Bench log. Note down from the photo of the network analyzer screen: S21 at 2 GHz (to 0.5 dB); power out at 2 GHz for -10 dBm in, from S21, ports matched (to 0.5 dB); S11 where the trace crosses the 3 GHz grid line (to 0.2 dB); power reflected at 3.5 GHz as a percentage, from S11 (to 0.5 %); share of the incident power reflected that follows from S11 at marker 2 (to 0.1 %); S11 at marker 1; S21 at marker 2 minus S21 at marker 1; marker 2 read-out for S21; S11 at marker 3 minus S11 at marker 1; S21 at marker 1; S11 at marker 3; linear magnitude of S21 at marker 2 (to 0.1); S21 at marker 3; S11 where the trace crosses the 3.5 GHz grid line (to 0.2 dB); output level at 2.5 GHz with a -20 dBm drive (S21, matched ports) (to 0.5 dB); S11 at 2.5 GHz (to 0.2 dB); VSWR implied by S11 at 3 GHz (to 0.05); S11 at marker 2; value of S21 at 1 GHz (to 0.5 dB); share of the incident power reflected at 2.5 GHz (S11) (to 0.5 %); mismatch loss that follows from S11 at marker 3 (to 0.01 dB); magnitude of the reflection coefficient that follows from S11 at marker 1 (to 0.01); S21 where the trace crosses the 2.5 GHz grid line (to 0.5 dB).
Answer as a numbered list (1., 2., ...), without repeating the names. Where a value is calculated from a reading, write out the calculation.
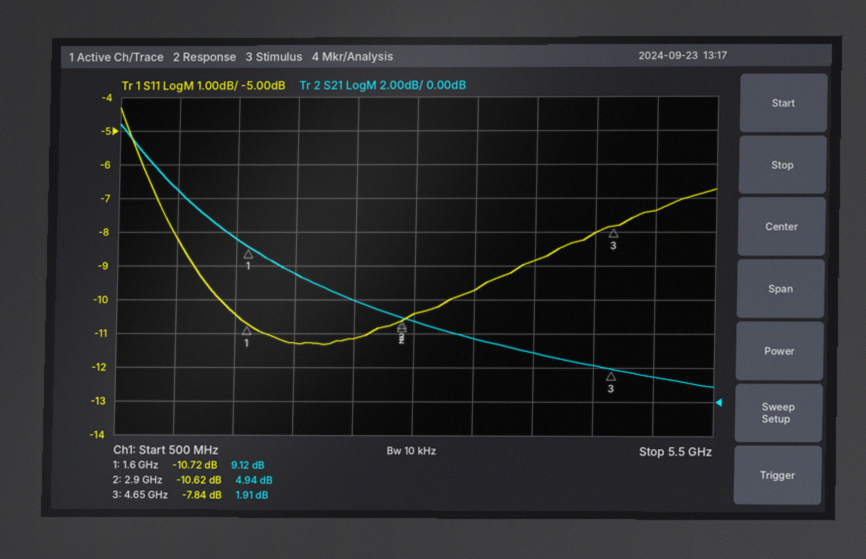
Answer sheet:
1. 7.5 dB
2. -10 dBm + (7.5 dB) = -2.5 dBm
3. -10.4 dB
4. 10^(-9.8/10) ≈ 10.5 %
5. 10^(-10.62/10) ≈ 8.7 %
6. -10.72 dB
7. 4.94 − (9.12) = -4.18 dB
8. 4.94 dB
9. -7.84 − (-10.72) = 2.88 dB
10. 9.12 dB
11. -7.84 dB
12. 10^(4.94/20) ≈ 1.8
13. 1.91 dB
14. -9.8 dB
15. -20 dBm + (6.0 dB) = -14.0 dBm
16. -11.2 dB
17. |Γ| = 10^(-10.4/20) = 0.3020; VSWR = (1 + 0.3020)/(1 − 0.3020) ≈ 1.87, so 1.85 to the nearest 0.05
18. -10.62 dB
19. 12.5 dB
20. 10^(-11.2/10) ≈ 7.59 %, so 7.5 % to the nearest 0.5 %
21. −10 log10(1 − 10^(-7.84/10)) ≈ 0.78 dB
22. 10^(-10.72/20) ≈ 0.29
23. 6.0 dB
